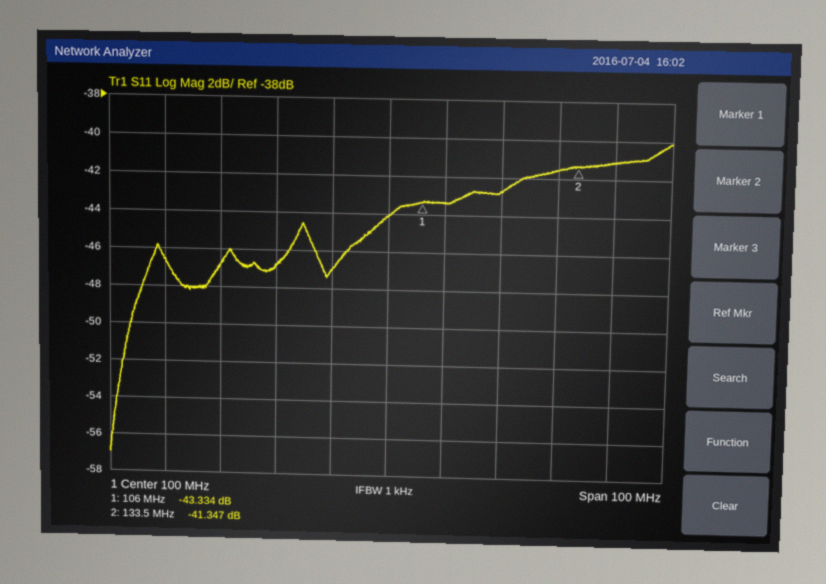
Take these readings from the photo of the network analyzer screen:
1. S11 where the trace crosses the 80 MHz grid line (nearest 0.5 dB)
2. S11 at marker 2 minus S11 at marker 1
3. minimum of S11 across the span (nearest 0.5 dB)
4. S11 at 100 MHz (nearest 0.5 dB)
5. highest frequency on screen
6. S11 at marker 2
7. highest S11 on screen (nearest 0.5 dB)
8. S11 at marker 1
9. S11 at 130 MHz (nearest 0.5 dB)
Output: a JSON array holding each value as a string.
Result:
["-47.0 dB", "1.987 dB", "-57.0 dB", "-44.0 dB", "150 MHz", "-41.347 dB", "-40.0 dB", "-43.334 dB", "-41.5 dB"]
